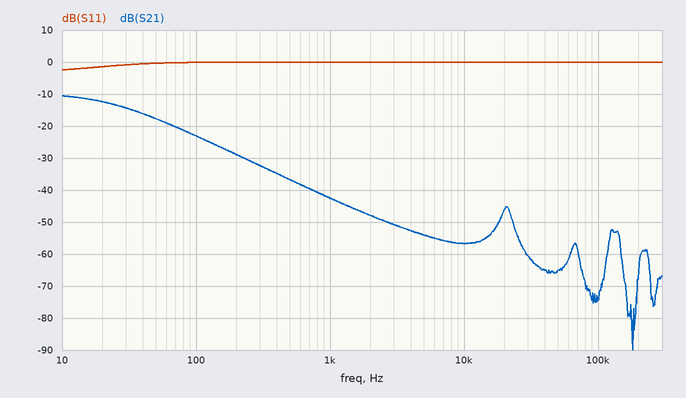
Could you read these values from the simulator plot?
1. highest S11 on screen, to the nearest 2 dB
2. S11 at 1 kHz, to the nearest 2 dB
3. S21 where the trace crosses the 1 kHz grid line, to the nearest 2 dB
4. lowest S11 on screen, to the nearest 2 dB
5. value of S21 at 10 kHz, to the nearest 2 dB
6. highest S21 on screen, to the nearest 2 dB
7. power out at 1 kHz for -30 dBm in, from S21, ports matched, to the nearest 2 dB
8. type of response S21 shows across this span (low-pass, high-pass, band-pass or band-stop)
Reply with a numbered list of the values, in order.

1. 0 dB
2. 0 dB
3. -42 dB
4. -2 dB
5. -56 dB
6. -10 dB
7. -72 dBm
8. low-pass
